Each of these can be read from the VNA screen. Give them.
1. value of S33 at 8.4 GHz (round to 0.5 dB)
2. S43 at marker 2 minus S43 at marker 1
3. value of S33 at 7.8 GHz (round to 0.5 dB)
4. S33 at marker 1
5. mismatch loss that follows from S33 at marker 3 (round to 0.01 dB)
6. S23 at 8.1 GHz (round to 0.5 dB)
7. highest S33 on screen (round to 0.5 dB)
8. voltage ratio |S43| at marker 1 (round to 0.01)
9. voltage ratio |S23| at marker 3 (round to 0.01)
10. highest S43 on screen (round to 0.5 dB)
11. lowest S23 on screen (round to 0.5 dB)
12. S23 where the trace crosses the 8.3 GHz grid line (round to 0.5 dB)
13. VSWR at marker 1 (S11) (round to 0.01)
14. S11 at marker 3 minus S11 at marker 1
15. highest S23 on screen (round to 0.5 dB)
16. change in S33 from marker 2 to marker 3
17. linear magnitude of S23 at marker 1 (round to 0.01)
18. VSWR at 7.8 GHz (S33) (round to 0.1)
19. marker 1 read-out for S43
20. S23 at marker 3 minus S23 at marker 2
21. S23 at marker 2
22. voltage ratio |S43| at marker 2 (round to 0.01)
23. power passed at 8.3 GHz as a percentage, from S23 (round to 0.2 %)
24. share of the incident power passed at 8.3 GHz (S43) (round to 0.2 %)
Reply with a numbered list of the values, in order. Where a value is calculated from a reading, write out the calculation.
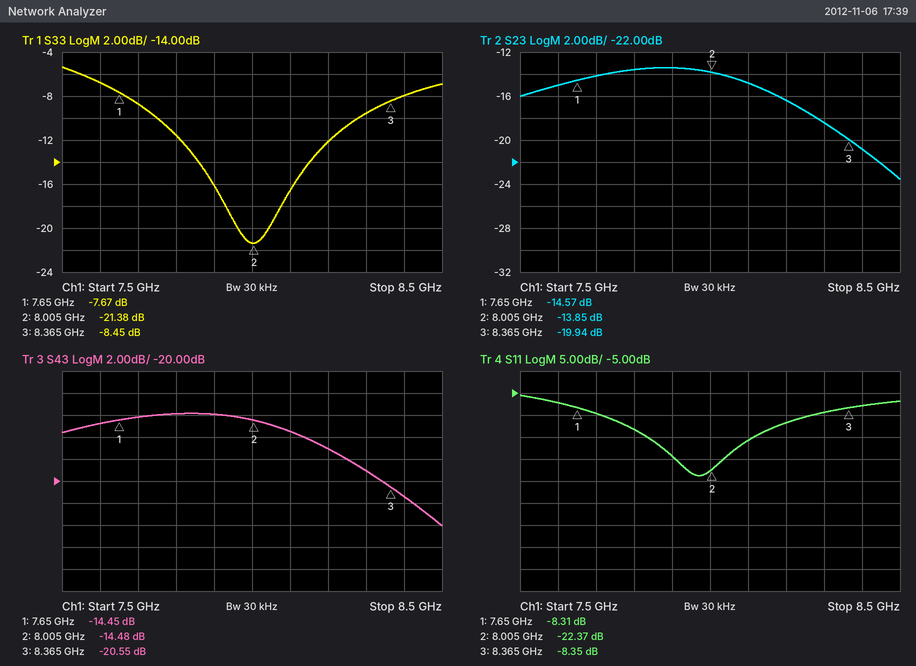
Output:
1. -8.0 dB
2. -14.48 − (-14.45) = -0.03 dB
3. -11.5 dB
4. -7.67 dB
5. −10 log10(1 − 10^(-8.45/10)) ≈ 0.67 dB
6. -15.0 dB
7. -5.5 dB
8. 10^(-14.45/20) ≈ 0.19
9. 10^(-19.94/20) ≈ 0.10
10. -14.0 dB
11. -23.5 dB
12. -18.5 dB
13. (1 + 0.3841)/(1 − 0.3841) ≈ 2.25
14. -8.35 − (-8.31) = -0.04 dB
15. -13.5 dB
16. -8.45 − (-21.38) = 12.93 dB
17. 10^(-14.57/20) ≈ 0.19
18. |Γ| = 10^(-11.5/20) = 0.2661; VSWR = (1 + 0.2661)/(1 − 0.2661) ≈ 1.7
19. -14.45 dB
20. -19.94 − (-13.85) = -6.09 dB
21. -13.85 dB
22. 10^(-14.48/20) ≈ 0.19
23. 10^(-18.5/10) ≈ 1.4 %
24. 10^(-19/10) ≈ 1.26 %, so 1.2 % to the nearest 0.2 %
